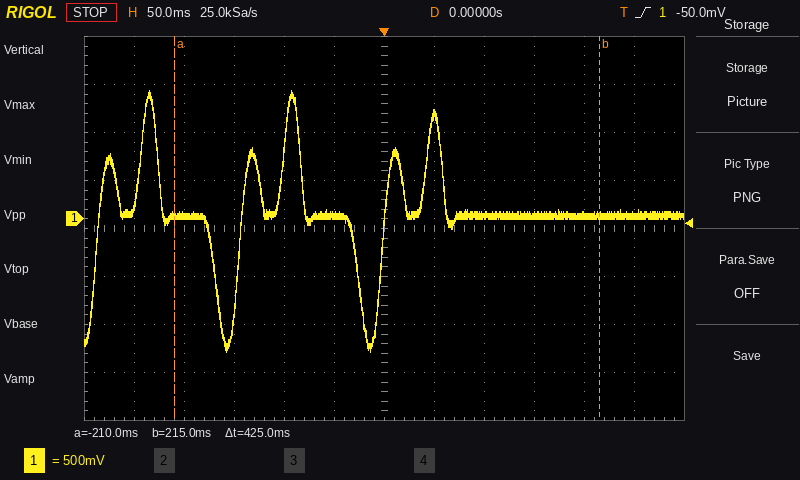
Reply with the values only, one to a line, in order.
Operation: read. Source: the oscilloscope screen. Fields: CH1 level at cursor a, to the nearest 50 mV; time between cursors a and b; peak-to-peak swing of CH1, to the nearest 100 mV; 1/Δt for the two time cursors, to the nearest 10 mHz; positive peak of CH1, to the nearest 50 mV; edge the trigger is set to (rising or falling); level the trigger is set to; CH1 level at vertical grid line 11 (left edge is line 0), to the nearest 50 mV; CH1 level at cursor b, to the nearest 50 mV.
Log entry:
50 mV
425 ms
2.70 V
2.35 Hz
1.35 V
rising
-50.0 mV
50 mV
50 mV
